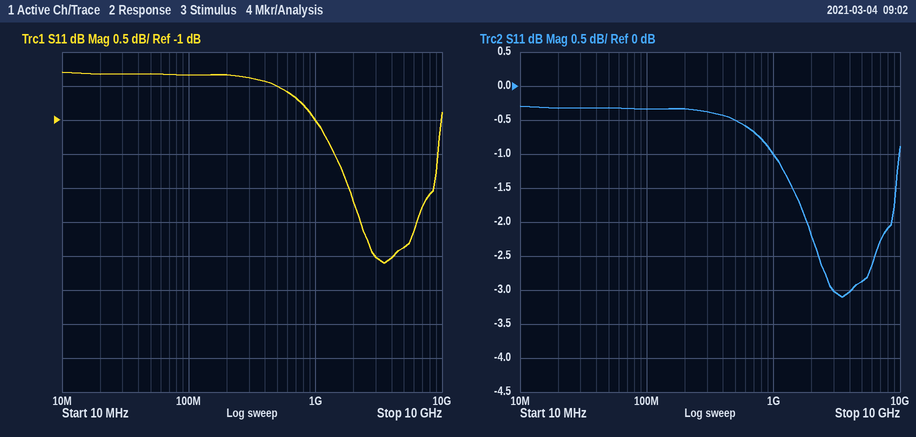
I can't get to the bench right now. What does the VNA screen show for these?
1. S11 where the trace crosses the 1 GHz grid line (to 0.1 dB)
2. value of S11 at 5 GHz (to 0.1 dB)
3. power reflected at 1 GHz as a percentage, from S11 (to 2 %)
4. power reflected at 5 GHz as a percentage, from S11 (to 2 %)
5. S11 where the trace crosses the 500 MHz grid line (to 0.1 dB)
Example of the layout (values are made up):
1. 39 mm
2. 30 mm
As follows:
1. -1.0 dB
2. -2.9 dB
3. 80 %
4. 52 %
5. -0.5 dB
